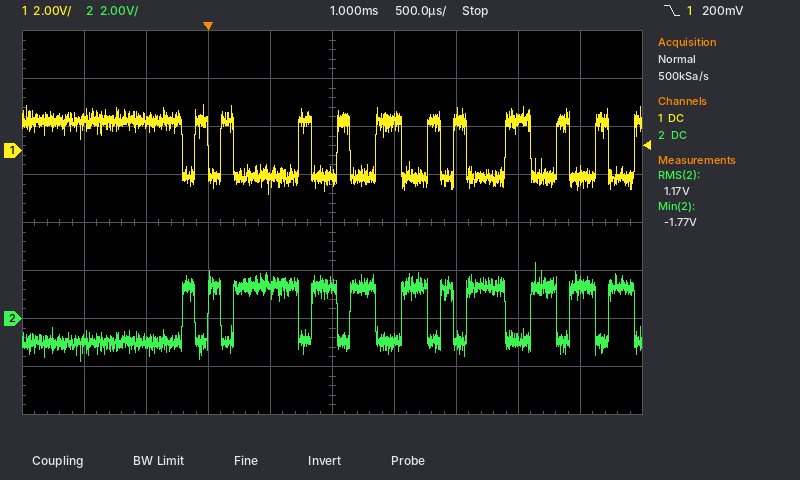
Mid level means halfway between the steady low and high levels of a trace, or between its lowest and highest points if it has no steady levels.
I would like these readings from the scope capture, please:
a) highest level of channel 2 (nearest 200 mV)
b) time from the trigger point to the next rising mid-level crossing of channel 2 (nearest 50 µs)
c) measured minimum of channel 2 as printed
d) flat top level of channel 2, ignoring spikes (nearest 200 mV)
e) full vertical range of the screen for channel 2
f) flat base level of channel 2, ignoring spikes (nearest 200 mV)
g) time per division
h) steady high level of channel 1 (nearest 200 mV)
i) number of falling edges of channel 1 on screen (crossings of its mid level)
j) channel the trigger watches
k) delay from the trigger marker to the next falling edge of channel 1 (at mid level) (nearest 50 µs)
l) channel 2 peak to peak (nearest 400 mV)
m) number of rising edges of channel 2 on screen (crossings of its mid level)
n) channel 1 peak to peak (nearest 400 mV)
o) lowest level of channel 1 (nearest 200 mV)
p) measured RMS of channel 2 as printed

2.4 V
200 µs
-1.77 V
1.4 V
16 V
-1.0 V
500 µs
1.2 V
11
channel 1
200 µs
4.0 V
11
3.6 V
-1.8 V
1.17 V
